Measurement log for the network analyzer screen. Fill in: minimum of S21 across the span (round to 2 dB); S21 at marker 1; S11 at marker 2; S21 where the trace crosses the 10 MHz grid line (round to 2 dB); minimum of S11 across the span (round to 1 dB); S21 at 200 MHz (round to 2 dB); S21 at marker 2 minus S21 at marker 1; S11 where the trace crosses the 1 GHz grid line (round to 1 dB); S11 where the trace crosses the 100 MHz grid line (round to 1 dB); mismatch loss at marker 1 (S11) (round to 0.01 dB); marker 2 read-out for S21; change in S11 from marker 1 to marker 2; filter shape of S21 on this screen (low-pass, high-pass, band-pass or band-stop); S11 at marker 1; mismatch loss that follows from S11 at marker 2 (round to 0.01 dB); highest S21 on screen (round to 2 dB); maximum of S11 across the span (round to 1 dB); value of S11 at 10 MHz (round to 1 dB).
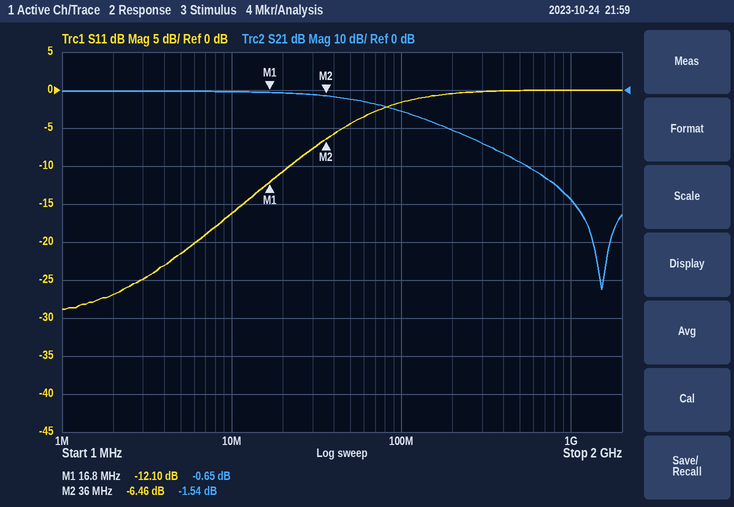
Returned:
-52 dB
-0.65 dB
-6.46 dB
0 dB
-29 dB
-10 dB
-0.89 dB
0 dB
-2 dB
0.28 dB
-1.54 dB
5.64 dB
low-pass
-12.10 dB
1.11 dB
0 dB
0 dB
-16 dB
